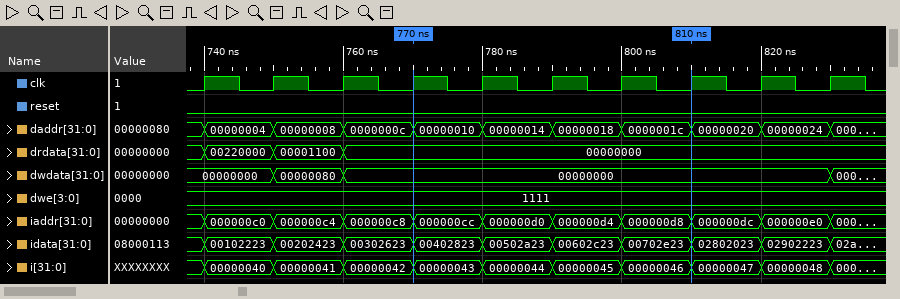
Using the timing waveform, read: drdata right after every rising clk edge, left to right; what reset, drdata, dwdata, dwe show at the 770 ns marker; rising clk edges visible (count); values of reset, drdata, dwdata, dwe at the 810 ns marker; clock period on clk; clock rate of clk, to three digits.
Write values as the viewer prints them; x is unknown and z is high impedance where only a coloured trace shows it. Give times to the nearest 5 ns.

00220000, 00001100, 00000000, 00000000, 00000000, 00000000, 00000000, 00000000, 00000000, 00000000
reset=0, drdata=00000000, dwdata=00000000, dwe=1111
10
reset=0, drdata=00000000, dwdata=00000000, dwe=1111
10 ns
100 MHz
